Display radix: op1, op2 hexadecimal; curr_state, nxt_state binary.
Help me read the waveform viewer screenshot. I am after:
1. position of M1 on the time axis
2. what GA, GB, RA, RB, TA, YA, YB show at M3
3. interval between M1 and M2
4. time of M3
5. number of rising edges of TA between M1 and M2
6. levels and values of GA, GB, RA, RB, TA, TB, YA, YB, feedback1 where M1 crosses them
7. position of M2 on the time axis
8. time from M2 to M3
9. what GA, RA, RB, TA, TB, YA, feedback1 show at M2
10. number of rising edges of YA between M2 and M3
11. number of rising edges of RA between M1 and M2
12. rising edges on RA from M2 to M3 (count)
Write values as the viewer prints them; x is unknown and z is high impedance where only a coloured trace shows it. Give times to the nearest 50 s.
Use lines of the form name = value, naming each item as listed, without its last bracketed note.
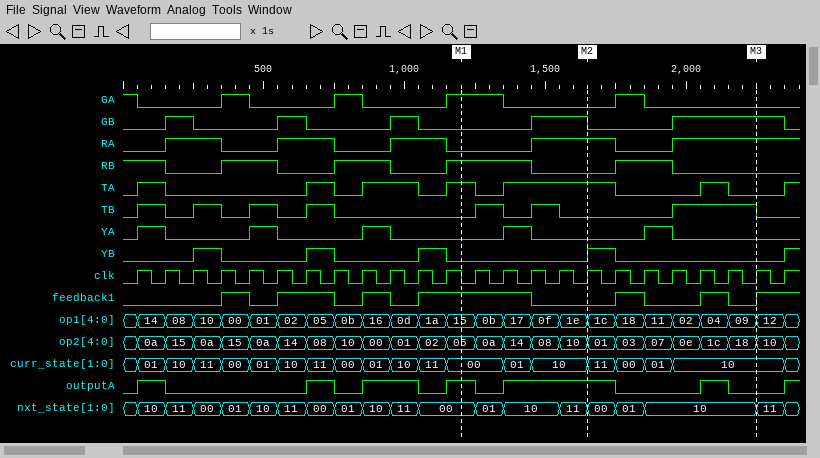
position of M1 on the time axis = 1200 s
what GA, GB, RA, RB, TA, YA, YB show at M3 = GA=0, GB=1, RA=1, RB=0, TA=0, YA=0, YB=0
interval between M1 and M2 = 450 s
time of M3 = 2250 s
number of rising edges of TA between M1 and M2 = 1
levels and values of GA, GB, RA, RB, TA, TB, YA, YB, feedback1 where M1 crosses them = GA=1, GB=0, RA=0, RB=1, TA=1, TB=0, YA=0, YB=0, feedback1=1
position of M2 on the time axis = 1650 s
time from M2 to M3 = 600 s
what GA, RA, RB, TA, TB, YA, feedback1 show at M2 = GA=0, RA=1, RB=0, TA=1, TB=0, YA=0, feedback1=0
number of rising edges of YA between M2 and M3 = 1
number of rising edges of RA between M1 and M2 = 1
rising edges on RA from M2 to M3 = 1
